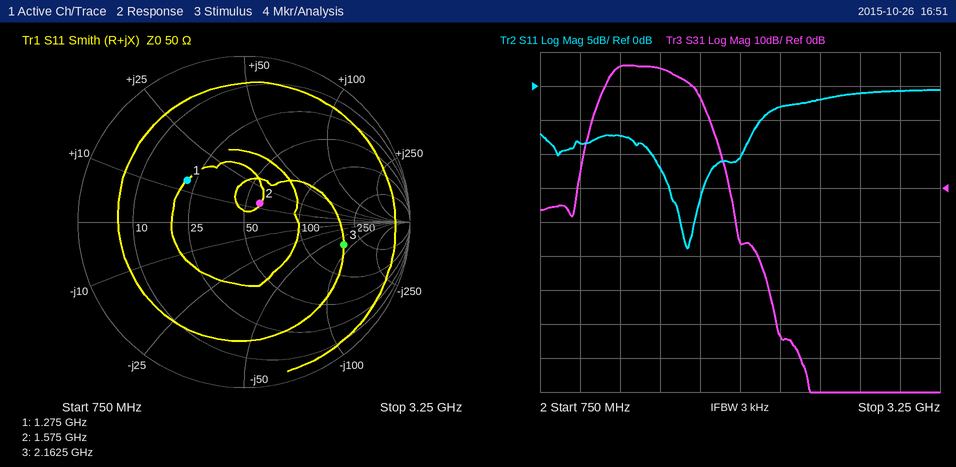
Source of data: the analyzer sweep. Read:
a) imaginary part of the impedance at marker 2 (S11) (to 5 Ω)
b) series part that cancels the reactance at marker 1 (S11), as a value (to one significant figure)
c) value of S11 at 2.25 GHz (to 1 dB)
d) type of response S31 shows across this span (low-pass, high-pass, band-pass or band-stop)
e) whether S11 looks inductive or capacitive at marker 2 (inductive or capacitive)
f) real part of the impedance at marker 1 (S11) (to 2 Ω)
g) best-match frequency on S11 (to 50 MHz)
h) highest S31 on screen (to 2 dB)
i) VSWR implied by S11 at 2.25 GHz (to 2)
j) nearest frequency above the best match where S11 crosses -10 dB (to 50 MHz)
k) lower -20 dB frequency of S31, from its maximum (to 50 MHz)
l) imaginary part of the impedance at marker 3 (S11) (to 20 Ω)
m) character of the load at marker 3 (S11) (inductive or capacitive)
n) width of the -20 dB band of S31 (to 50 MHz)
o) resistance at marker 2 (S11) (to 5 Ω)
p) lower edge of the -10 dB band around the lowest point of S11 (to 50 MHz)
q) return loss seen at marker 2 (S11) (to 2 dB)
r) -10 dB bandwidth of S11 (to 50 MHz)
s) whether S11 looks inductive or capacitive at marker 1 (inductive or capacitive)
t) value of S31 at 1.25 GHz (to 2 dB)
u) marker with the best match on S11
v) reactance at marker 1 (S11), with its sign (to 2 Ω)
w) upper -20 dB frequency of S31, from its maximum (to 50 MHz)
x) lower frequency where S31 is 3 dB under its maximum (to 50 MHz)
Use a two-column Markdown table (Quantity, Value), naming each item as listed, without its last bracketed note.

| Quantity | Value |
|---|---|
| imaginary part of the impedance at marker 2 (S11) | +15 Ω |
| series part that cancels the reactance at marker 1 (S11), as a value | 9 pF |
| value of S11 at 2.25 GHz | -3 dB |
| type of response S31 shows across this span | band-pass |
| whether S11 looks inductive or capacitive at marker 2 | inductive |
| real part of the impedance at marker 1 (S11) | 22 Ω |
| best-match frequency on S11 | 1.65 GHz |
| highest S31 on screen | 36 dB |
| VSWR implied by S11 at 2.25 GHz | 6 |
| nearest frequency above the best match where S11 crosses -10 dB | 2.00 GHz |
| lower -20 dB frequency of S31, from its maximum | 1.05 GHz |
| imaginary part of the impedance at marker 3 (S11) | -80 Ω |
| character of the load at marker 3 (S11) | capacitive |
| width of the -20 dB band of S31 | 800 MHz |
| resistance at marker 2 (S11) | 60 Ω |
| lower edge of the -10 dB band around the lowest point of S11 | 1.45 GHz |
| return loss seen at marker 2 (S11) | 16 dB |
| -10 dB bandwidth of S11 | 550 MHz |
| whether S11 looks inductive or capacitive at marker 1 | inductive |
| value of S31 at 1.25 GHz | 36 dB |
| marker with the best match on S11 | marker 2 |
| reactance at marker 1 (S11), with its sign | +14 Ω |
| upper -20 dB frequency of S31, from its maximum | 1.85 GHz |
| lower frequency where S31 is 3 dB under its maximum | 1.20 GHz |
